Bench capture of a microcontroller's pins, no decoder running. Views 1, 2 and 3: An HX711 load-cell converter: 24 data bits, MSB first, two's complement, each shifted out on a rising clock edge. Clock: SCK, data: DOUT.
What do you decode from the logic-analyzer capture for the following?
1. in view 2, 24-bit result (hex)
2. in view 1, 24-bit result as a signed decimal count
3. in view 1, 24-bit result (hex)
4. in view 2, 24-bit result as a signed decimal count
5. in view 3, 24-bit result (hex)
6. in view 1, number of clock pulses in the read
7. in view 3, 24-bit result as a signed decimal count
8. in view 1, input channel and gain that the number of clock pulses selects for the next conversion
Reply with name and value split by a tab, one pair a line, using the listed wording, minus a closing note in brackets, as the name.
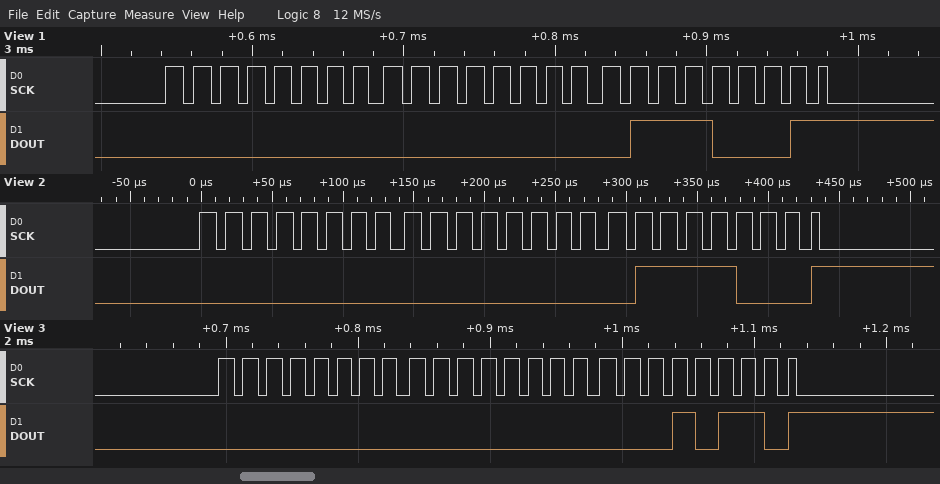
in view 2, 24-bit result	0x000078
in view 1, 24-bit result as a signed decimal count	113
in view 1, 24-bit result	0x000071
in view 2, 24-bit result as a signed decimal count	120
in view 3, 24-bit result	0x000016
in view 1, number of clock pulses in the read	25
in view 3, 24-bit result as a signed decimal count	22
in view 1, input channel and gain that the number of clock pulses selects for the next conversion	channel A, gain 128
